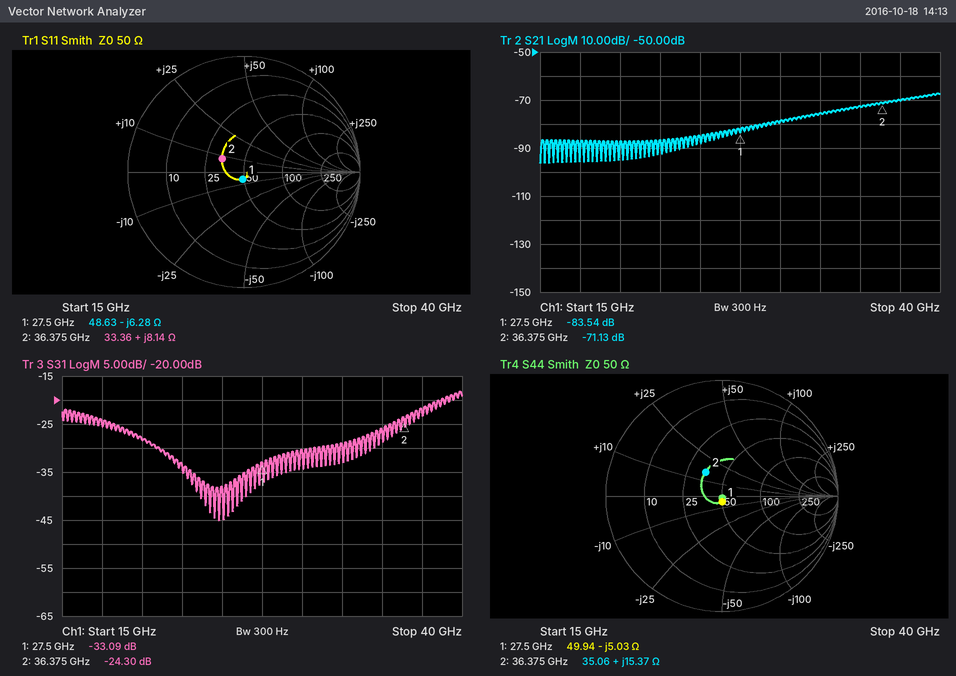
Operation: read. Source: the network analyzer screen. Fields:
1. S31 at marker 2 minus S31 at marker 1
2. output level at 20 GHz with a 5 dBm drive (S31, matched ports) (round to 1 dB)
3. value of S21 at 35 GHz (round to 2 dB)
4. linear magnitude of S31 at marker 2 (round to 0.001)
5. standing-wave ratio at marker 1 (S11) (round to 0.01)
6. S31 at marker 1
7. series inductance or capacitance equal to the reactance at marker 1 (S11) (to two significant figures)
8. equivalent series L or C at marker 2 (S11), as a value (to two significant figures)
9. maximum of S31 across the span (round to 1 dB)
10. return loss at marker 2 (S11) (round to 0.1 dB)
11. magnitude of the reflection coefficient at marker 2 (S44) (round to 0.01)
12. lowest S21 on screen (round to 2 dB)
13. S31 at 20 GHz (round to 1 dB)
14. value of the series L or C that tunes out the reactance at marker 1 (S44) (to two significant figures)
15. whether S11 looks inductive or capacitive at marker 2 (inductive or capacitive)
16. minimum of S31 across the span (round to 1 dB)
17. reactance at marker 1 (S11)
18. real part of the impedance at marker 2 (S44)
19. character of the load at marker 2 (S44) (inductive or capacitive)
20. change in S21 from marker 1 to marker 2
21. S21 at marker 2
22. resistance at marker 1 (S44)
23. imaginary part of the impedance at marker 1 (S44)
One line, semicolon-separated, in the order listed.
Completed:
8.79 dB; -23 dBm; -72 dB; 0.061; 1.14; -33.09 dB; 920 fF; 36 pH; -18 dB; 13.1 dB; 0.25; -96 dB; -28 dB; 29 pH; inductive; -45 dB; -6.28 Ω; 35.06 Ω; inductive; 12.41 dB; -71.13 dB; 49.94 Ω; -5.03 Ω
